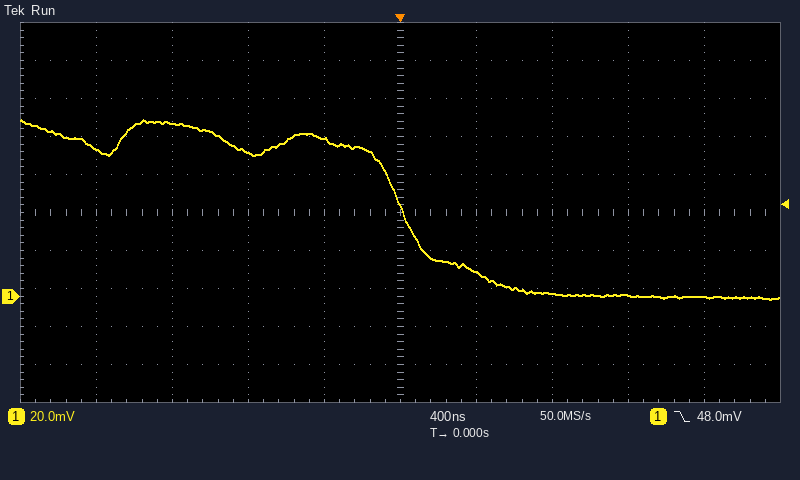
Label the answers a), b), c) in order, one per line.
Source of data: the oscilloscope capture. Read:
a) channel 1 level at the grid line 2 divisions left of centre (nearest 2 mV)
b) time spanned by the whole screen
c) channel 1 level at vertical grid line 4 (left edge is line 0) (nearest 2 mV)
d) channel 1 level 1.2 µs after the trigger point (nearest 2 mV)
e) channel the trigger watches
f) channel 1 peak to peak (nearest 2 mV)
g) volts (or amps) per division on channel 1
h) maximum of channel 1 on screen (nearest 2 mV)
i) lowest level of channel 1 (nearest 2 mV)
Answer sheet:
a) 76 mV
b) 4 µs
c) 82 mV
d) 0 mV
e) channel 1
f) 94 mV
g) 20 mV
h) 92 mV
i) -2 mV
